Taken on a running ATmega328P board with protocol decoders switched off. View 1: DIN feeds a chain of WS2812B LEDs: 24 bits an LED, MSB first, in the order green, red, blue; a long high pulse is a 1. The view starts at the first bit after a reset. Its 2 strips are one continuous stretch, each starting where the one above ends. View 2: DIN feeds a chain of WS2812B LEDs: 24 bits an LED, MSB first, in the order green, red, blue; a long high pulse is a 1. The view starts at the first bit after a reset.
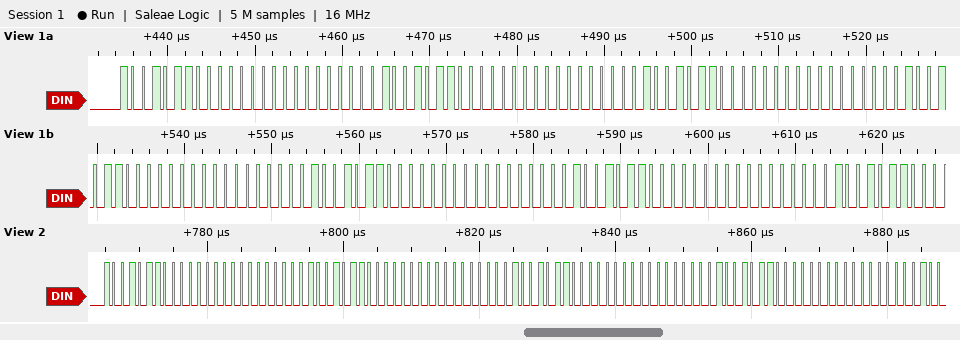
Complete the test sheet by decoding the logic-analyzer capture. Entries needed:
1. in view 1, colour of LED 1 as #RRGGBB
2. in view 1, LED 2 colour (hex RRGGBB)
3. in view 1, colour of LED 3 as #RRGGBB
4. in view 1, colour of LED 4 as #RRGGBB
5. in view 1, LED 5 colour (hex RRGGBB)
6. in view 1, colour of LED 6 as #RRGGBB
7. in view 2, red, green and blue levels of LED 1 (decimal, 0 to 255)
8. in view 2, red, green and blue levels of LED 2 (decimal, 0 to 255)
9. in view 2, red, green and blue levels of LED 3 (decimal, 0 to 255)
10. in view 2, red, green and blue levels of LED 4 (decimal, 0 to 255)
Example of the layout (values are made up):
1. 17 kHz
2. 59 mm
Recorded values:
1. #009600
2. #009600
3. #009600
4. #009600
5. #009600
6. #009600
7. 0, 150, 0
8. 0, 150, 0
9. 0, 150, 0
10. 0, 150, 0
